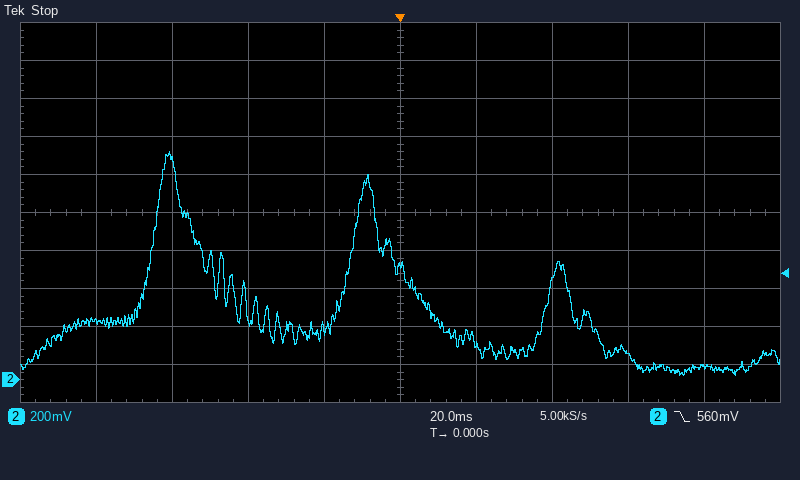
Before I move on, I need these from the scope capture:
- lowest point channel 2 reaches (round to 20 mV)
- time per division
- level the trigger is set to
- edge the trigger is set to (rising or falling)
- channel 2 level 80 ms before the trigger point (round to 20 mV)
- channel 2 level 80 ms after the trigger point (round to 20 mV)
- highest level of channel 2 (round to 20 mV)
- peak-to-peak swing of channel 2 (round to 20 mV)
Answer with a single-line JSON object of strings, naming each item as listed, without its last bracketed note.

{"lowest point channel 2 reaches": "20 mV", "time per division": "20 ms", "level the trigger is set to": "560 mV", "edge the trigger is set to": "falling", "channel 2 level 80 ms before the trigger point": "300 mV", "channel 2 level 80 ms after the trigger point": "60 mV", "highest level of channel 2": "1.20 V", "peak-to-peak swing of channel 2": "1.18 V"}
